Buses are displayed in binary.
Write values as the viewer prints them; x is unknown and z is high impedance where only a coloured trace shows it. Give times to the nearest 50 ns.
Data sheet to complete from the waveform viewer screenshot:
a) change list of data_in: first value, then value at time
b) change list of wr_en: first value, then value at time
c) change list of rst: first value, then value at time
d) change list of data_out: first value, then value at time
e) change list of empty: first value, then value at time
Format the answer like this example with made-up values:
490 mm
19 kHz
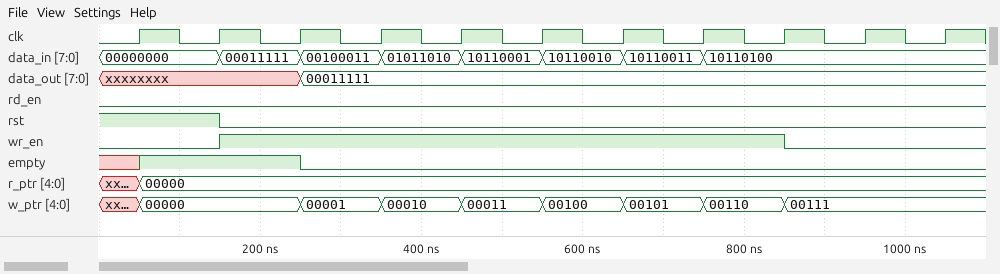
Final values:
00000000, 00011111 at 150 ns, 00100011 at 250 ns, 01011010 at 350 ns, 10110001 at 450 ns, 10110010 at 550 ns, 10110011 at 650 ns, 10110100 at 750 ns
0, 1 at 150 ns, 0 at 850 ns
1, 0 at 150 ns
xxxxxxxx, 00011111 at 250 ns
x, 1 at 50 ns, 0 at 250 ns
